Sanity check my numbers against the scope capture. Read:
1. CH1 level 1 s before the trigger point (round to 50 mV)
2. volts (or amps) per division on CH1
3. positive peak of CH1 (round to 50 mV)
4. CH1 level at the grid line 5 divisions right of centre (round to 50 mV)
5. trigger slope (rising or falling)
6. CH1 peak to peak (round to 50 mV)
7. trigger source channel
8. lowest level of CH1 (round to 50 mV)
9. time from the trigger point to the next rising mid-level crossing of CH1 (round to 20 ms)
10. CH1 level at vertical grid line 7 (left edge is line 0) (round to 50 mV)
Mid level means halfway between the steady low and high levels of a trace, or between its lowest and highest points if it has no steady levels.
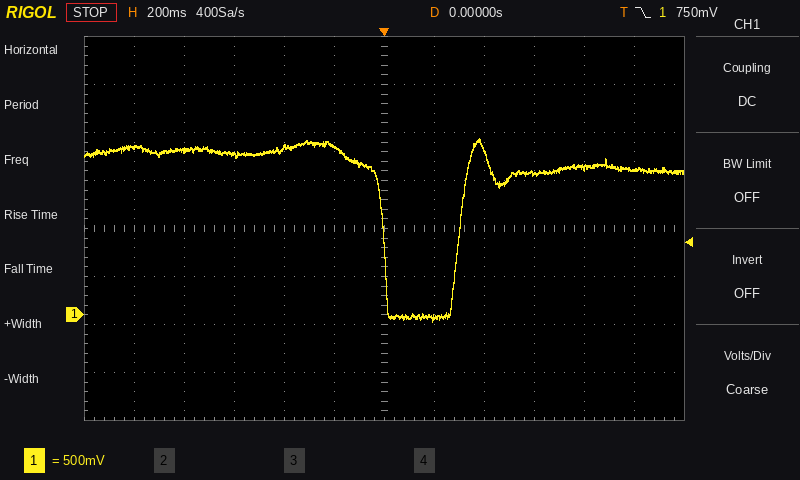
1.75 V
500 mV
1.85 V
1.50 V
falling
1.90 V
CH1
-50 mV
300 ms
-50 mV
